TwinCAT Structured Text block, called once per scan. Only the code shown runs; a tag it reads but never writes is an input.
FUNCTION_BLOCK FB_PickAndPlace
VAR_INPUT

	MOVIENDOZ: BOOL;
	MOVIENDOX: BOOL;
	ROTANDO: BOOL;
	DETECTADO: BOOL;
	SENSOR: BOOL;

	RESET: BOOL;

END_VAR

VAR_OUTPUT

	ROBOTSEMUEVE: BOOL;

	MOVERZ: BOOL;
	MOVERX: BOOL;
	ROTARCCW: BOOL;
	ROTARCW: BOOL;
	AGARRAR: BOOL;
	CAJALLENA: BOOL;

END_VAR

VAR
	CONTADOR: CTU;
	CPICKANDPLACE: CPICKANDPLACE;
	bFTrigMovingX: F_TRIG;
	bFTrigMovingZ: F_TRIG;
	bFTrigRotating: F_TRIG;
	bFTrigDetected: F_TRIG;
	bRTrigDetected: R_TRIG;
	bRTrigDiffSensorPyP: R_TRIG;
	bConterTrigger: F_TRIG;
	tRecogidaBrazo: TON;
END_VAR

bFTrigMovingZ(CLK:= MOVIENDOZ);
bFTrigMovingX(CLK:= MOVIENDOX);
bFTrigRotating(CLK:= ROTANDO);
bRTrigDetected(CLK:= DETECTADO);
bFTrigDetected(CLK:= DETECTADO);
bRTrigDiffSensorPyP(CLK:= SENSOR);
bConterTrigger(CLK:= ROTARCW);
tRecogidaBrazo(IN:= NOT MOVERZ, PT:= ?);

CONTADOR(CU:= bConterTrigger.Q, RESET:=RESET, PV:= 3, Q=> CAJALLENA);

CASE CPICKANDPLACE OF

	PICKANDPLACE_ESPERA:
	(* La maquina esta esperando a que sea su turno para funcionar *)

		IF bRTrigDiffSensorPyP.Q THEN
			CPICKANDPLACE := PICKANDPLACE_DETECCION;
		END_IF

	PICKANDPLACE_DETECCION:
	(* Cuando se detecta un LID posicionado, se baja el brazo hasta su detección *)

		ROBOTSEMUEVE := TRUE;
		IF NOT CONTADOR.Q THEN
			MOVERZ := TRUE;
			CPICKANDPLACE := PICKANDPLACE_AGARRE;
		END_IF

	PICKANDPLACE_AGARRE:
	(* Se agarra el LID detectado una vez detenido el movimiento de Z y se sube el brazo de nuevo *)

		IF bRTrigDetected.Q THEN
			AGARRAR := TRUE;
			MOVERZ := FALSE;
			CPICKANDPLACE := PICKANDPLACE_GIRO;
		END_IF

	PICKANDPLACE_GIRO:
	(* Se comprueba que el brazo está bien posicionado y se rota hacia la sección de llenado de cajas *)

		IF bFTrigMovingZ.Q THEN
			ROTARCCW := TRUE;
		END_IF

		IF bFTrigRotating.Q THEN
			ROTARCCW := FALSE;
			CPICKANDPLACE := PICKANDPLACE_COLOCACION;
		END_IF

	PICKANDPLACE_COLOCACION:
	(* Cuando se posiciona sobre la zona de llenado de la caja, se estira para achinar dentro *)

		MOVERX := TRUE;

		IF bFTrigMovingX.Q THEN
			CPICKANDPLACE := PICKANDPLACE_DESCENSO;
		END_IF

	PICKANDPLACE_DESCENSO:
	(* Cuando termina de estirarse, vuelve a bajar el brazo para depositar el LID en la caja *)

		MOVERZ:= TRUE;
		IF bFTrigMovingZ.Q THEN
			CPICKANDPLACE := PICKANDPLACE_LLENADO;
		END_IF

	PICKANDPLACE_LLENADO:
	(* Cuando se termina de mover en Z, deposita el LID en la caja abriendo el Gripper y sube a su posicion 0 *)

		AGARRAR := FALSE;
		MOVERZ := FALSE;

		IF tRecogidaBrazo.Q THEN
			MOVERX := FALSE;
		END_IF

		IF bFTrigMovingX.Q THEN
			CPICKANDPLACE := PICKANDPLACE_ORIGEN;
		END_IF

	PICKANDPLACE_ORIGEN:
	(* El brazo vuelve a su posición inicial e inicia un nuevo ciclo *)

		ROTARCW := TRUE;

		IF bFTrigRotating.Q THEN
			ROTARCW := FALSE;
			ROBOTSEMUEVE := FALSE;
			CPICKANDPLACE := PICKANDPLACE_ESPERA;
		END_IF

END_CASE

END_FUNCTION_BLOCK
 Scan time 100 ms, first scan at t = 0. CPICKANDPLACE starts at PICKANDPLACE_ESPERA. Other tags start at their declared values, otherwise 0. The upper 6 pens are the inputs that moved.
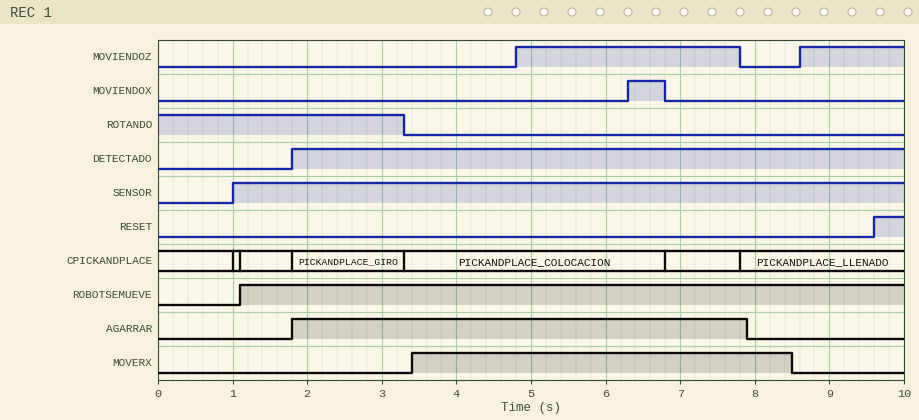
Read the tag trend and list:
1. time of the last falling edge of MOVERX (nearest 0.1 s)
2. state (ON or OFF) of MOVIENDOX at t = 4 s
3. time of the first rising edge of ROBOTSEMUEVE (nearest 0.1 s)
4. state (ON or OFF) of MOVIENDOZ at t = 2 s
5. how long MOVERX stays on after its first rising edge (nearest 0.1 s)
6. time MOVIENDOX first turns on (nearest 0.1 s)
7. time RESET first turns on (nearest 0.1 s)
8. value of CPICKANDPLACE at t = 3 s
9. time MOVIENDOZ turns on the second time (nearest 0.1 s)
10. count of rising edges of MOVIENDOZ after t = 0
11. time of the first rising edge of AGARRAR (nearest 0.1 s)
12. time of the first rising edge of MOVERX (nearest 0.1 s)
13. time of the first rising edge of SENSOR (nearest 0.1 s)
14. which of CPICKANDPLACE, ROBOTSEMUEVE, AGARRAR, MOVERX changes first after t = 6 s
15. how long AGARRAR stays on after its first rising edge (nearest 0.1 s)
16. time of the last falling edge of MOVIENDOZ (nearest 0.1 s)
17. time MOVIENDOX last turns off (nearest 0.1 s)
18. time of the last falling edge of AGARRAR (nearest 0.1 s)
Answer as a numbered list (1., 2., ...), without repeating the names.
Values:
1. 8.5 s
2. OFF
3. 1.1 s
4. OFF
5. 5.1 s
6. 6.3 s
7. 9.6 s
8. PICKANDPLACE_GIRO
9. 8.6 s
10. 2
11. 1.8 s
12. 3.4 s
13. 1.0 s
14. CPICKANDPLACE
15. 6.1 s
16. 7.8 s
17. 6.8 s
18. 7.9 s
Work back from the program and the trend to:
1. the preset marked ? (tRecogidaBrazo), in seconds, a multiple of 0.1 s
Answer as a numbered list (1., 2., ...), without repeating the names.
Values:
1. 0.5 s
